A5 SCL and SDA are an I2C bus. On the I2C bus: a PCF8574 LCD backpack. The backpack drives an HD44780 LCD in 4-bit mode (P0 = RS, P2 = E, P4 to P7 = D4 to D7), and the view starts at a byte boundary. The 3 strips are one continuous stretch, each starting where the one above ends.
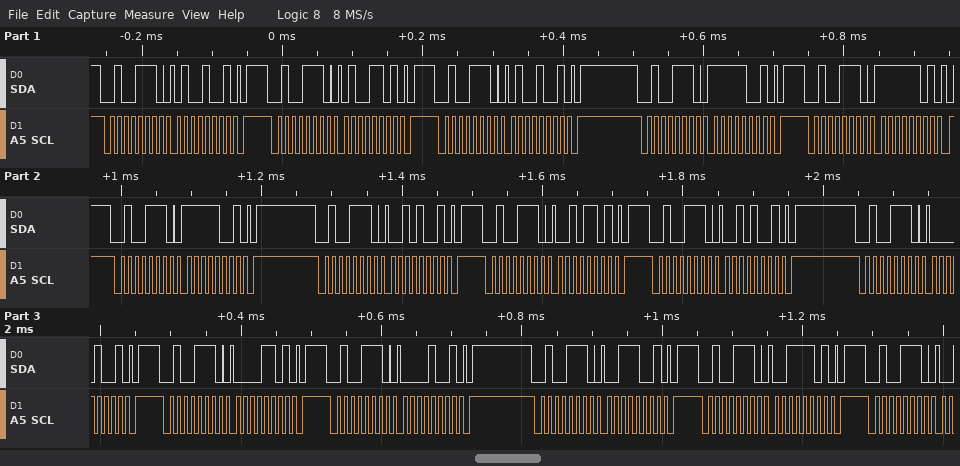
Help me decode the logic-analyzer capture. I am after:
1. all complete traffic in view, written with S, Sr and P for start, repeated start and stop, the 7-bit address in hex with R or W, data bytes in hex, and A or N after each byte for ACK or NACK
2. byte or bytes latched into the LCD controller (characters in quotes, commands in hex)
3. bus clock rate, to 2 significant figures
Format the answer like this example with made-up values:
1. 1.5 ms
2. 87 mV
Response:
1. S 27W A 49 A P S 27W A 4D A P S 27W A 49 A P S 27W A F9 A P S 27W A FD A P S 27W A F9 A P S 27W A 29 A P S 27W A 2D A P S 27W A 29 A P S 27W A 09 A P S 27W A 0D A P S 27W A 09 A P S 27W A 39 A P S 27W A 3D A P S 27W A
2. 'O' ' '
3. 100 kHz
